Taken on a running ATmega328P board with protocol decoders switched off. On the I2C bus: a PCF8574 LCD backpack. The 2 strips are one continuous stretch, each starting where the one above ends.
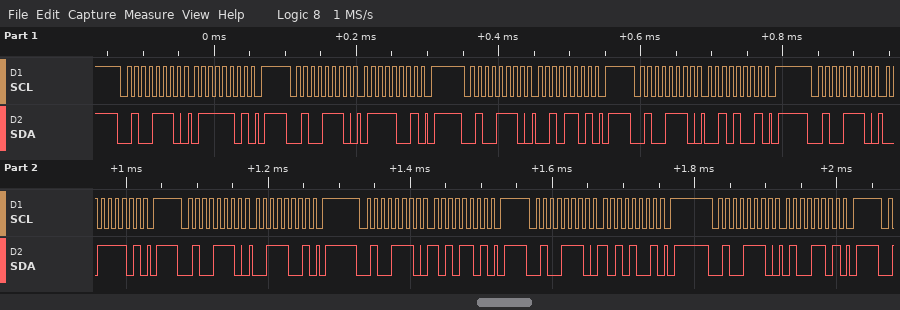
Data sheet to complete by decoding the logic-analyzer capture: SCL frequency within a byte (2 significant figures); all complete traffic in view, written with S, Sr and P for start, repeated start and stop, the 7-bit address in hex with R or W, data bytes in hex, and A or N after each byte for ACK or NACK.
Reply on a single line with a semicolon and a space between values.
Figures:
100 kHz; S 27W A 7D A P S 27W A 79 A P S 27W A 2D A P S 27W A 29 A P S 27W A 3D A P S 27W A 39 A P S 27W A AD A P S 27W A A9 A P S 27W A 4D A P
